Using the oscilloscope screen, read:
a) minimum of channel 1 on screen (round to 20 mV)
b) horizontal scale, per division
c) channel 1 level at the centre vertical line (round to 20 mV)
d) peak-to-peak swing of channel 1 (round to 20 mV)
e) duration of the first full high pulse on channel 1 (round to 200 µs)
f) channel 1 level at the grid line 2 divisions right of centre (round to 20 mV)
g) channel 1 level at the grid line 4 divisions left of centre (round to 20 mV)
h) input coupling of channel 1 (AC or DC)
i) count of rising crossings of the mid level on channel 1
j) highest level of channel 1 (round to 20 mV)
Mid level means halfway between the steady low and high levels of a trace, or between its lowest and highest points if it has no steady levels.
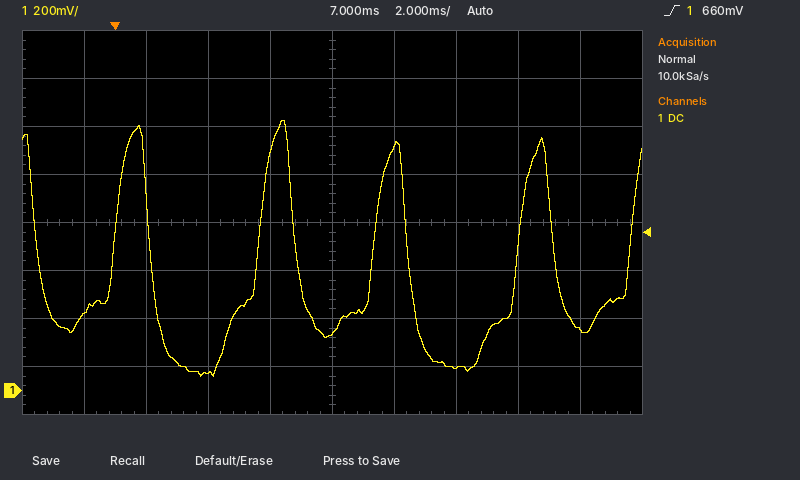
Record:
60 mV
2 ms
240 mV
1.06 V
1.2 ms
100 mV
320 mV
DC
5
1.12 V
